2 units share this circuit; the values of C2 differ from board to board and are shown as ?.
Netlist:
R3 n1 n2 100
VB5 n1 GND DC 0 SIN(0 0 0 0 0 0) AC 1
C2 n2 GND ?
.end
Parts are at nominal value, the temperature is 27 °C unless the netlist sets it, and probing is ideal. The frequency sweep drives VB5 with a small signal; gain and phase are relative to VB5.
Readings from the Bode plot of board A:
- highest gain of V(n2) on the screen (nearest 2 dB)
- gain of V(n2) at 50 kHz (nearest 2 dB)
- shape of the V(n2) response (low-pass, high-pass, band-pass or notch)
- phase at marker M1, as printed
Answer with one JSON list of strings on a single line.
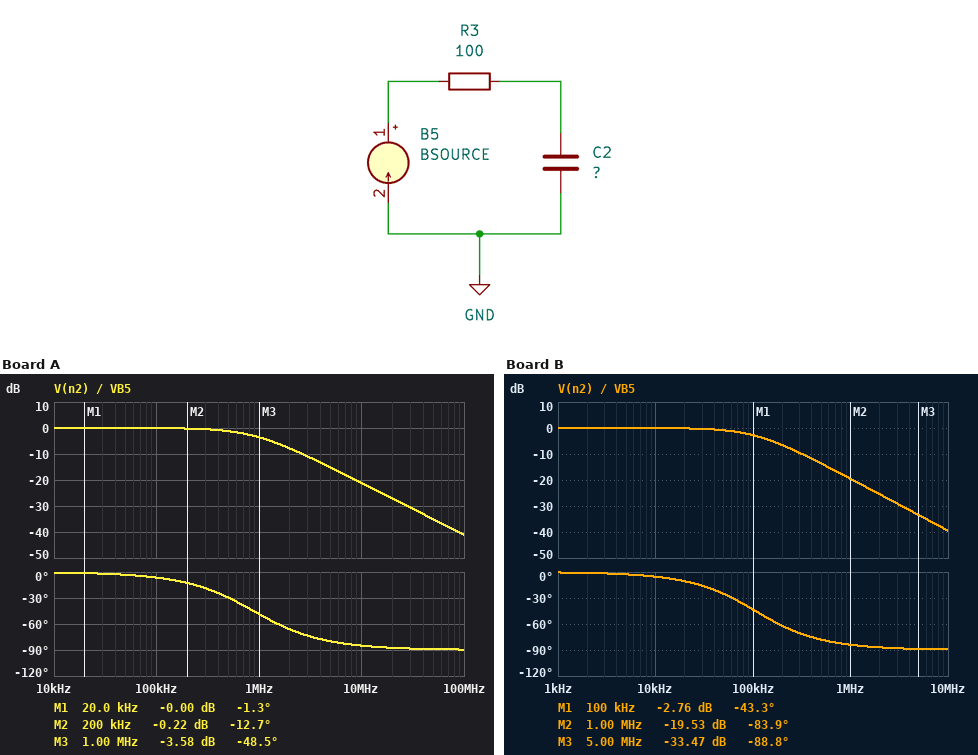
["0 dB", "0 dB", "low-pass", "-1.3 deg"]
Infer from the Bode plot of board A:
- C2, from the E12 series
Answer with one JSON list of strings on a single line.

["1.8 nF"]
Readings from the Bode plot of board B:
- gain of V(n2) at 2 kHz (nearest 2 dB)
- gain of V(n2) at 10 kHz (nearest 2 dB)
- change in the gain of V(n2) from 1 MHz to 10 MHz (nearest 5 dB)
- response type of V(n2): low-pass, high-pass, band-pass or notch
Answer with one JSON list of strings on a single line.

["0 dB", "0 dB", "-20 dB", "low-pass"]
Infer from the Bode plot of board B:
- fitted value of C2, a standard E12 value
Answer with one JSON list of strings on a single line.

["15 nF"]
